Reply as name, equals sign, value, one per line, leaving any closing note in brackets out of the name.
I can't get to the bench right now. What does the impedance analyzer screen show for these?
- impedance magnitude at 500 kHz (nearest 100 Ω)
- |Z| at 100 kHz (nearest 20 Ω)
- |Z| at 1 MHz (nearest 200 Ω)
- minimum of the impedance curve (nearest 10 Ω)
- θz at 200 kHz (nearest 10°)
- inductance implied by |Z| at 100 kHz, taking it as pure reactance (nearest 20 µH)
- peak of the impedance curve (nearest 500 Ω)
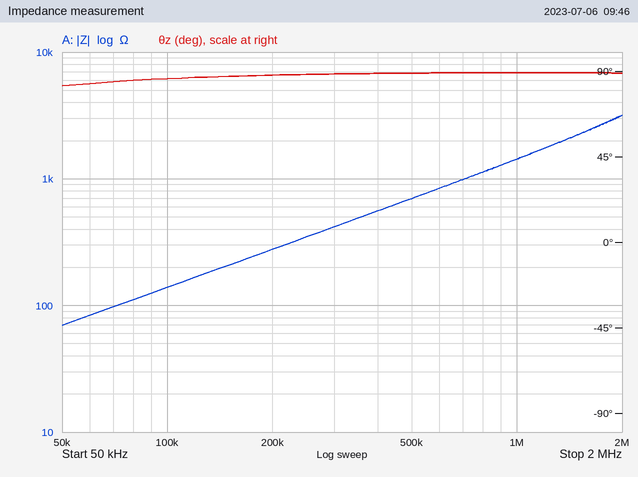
impedance magnitude at 500 kHz = 700 Ω
|Z| at 100 kHz = 140 Ω
|Z| at 1 MHz = 1.4 kΩ
minimum of the impedance curve = 70 Ω
θz at 200 kHz = 90°
inductance implied by |Z| at 100 kHz, taking it as pure reactance = 220 µH
peak of the impedance curve = 3.0 kΩ
